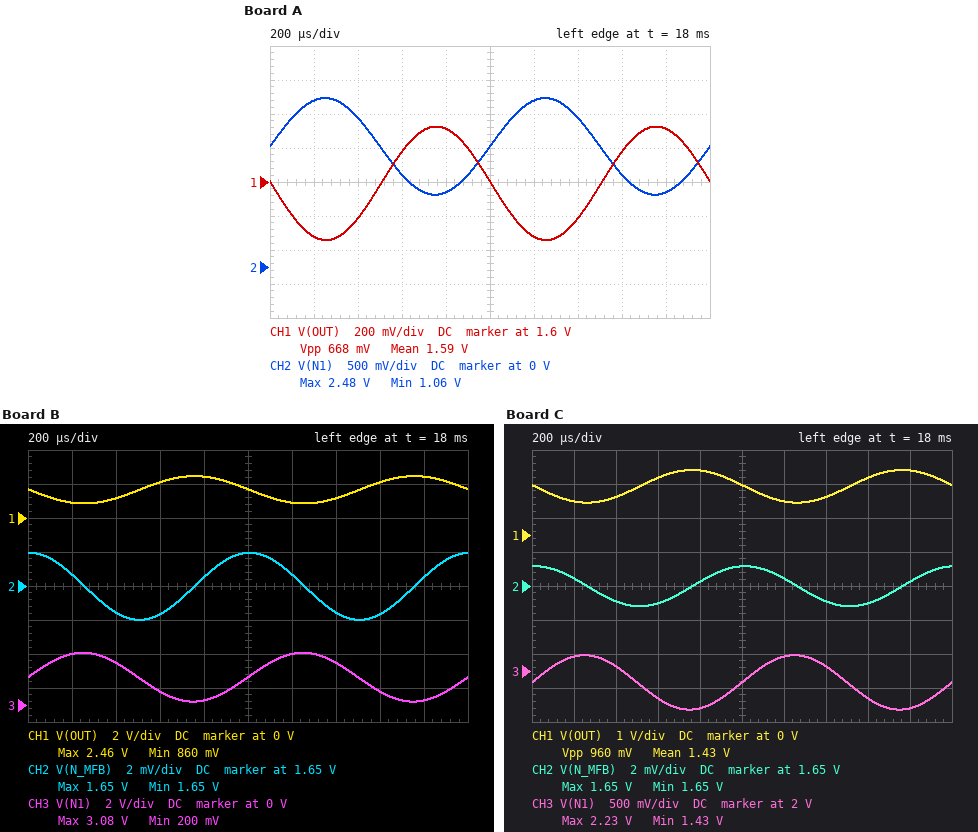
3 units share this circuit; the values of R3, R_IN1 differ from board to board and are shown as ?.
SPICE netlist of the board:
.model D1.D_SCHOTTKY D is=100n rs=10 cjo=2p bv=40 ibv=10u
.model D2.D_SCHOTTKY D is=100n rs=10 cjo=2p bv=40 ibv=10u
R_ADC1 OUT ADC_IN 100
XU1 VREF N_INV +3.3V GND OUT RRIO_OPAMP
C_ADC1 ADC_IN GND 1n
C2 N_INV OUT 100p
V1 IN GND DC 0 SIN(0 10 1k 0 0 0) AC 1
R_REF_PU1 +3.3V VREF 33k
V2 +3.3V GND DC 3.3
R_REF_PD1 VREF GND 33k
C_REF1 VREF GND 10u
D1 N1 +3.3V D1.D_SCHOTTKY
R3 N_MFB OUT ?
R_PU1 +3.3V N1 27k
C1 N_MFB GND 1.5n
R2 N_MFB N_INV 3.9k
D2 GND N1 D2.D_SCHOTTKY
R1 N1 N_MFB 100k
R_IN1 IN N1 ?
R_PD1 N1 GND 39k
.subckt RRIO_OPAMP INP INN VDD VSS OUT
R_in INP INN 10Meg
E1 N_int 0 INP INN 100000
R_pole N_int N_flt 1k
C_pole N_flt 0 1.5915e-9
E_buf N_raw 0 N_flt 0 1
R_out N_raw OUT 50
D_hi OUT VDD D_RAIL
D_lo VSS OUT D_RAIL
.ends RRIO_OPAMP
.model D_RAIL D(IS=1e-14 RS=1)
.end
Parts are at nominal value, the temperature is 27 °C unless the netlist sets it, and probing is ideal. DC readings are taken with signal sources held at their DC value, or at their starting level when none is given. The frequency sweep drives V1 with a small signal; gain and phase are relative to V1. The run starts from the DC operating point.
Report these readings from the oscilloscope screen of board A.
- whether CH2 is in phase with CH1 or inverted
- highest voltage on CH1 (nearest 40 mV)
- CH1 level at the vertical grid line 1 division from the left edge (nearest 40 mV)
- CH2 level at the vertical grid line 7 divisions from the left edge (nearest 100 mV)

inverted
1.92 V
1.28 V
2.2 V
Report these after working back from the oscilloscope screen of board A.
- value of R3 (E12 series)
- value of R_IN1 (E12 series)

47 kΩ
180 kΩ
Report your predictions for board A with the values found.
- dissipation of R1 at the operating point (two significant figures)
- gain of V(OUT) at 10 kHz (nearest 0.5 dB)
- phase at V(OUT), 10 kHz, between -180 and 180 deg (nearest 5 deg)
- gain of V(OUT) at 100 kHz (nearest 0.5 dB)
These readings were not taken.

150 nW
-29.0 dB
160 deg
-50.0 dB
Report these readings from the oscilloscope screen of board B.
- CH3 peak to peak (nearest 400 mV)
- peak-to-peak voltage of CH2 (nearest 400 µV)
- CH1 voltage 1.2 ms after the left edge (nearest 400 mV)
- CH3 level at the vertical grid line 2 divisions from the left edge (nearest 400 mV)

2.8 V
4.0 mV
800 mV
2.4 V
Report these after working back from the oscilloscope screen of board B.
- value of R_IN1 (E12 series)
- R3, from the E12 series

82 kΩ
56 kΩ
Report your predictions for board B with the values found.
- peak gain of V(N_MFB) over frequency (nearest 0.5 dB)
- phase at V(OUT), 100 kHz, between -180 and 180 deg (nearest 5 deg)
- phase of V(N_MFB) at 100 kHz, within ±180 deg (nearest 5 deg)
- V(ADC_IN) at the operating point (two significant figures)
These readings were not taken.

-46.0 dB
15 deg
-75 deg
1.7 V
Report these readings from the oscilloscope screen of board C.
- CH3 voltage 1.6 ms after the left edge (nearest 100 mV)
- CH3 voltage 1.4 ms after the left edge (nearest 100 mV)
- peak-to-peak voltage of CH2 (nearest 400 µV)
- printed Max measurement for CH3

1.6 V
2.1 V
2.4 mV
2.23 V
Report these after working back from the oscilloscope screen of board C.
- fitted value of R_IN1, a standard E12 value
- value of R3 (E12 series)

330 kΩ
120 kΩ
